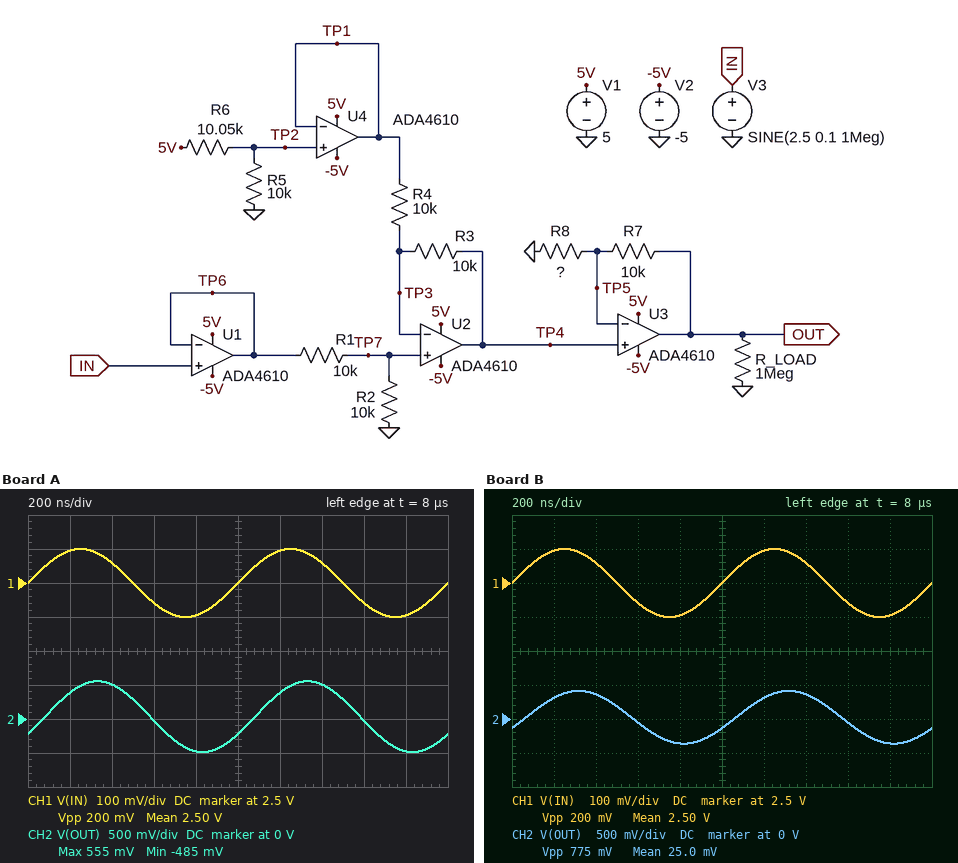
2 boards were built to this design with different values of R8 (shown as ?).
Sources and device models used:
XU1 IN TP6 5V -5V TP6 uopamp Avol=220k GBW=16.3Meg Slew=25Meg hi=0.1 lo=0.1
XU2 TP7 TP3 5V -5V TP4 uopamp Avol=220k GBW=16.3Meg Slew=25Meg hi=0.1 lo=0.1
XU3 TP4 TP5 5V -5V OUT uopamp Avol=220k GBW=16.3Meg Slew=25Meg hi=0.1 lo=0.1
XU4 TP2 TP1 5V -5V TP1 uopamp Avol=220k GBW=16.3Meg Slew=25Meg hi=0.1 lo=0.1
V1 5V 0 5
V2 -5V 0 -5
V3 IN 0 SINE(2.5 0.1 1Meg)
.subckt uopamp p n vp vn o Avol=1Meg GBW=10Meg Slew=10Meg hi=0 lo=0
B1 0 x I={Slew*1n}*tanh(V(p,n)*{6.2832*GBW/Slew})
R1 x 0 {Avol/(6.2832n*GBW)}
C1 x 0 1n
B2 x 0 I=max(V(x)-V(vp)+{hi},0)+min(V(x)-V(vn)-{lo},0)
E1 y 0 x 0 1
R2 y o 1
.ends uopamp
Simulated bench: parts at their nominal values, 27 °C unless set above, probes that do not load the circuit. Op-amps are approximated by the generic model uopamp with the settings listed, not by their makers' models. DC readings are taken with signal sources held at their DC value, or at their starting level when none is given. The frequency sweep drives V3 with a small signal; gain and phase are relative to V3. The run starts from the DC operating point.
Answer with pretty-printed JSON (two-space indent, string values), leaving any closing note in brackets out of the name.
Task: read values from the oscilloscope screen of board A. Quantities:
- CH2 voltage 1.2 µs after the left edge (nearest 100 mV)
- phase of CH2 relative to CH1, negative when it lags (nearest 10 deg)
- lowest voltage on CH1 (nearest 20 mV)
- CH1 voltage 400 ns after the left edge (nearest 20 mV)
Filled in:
{
  "CH2 voltage 1.2 µs after the left edge": "400 mV",
  "phase of CH2 relative to CH1, negative when it lags": "-30 deg",
  "lowest voltage on CH1": "2.40 V",
  "CH1 voltage 400 ns after the left edge": "2.56 V"
}
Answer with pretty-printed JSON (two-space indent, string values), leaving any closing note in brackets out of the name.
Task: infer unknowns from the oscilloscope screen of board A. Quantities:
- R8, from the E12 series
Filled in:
{
  "R8, from the E12 series": "2.2 kΩ"
}
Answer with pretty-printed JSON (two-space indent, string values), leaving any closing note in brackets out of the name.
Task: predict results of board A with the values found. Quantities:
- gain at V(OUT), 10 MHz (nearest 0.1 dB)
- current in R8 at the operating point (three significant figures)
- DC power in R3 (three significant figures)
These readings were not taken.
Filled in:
{
  "gain at V(OUT), 10 MHz": "-1.5 dB",
  "current in R8 at the operating point": "2.83 µA",
  "DC power in R3": "155 µW"
}
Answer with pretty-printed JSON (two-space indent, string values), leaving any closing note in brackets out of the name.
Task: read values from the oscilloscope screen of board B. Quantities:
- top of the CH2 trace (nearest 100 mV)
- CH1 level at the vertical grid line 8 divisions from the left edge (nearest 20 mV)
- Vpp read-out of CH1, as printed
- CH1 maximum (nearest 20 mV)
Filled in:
{
  "top of the CH2 trace": "400 mV",
  "CH1 level at the vertical grid line 8 divisions from the left edge": "2.44 V",
  "Vpp read-out of CH1, as printed": "200 mV",
  "CH1 maximum": "2.60 V"
}
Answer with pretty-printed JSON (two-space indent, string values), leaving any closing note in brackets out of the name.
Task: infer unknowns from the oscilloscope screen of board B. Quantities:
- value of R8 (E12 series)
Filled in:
{
  "value of R8": "3.3 kΩ"
}
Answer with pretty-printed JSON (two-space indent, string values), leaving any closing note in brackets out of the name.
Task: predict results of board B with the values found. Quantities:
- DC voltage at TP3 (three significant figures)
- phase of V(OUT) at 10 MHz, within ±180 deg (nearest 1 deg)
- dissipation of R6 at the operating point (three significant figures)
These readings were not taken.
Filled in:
{
  "DC voltage at TP3": "1.25 V",
  "phase of V(OUT) at 10 MHz, within ±180 deg": "-150 deg",
  "dissipation of R6 at the operating point": "625 µW"
}
